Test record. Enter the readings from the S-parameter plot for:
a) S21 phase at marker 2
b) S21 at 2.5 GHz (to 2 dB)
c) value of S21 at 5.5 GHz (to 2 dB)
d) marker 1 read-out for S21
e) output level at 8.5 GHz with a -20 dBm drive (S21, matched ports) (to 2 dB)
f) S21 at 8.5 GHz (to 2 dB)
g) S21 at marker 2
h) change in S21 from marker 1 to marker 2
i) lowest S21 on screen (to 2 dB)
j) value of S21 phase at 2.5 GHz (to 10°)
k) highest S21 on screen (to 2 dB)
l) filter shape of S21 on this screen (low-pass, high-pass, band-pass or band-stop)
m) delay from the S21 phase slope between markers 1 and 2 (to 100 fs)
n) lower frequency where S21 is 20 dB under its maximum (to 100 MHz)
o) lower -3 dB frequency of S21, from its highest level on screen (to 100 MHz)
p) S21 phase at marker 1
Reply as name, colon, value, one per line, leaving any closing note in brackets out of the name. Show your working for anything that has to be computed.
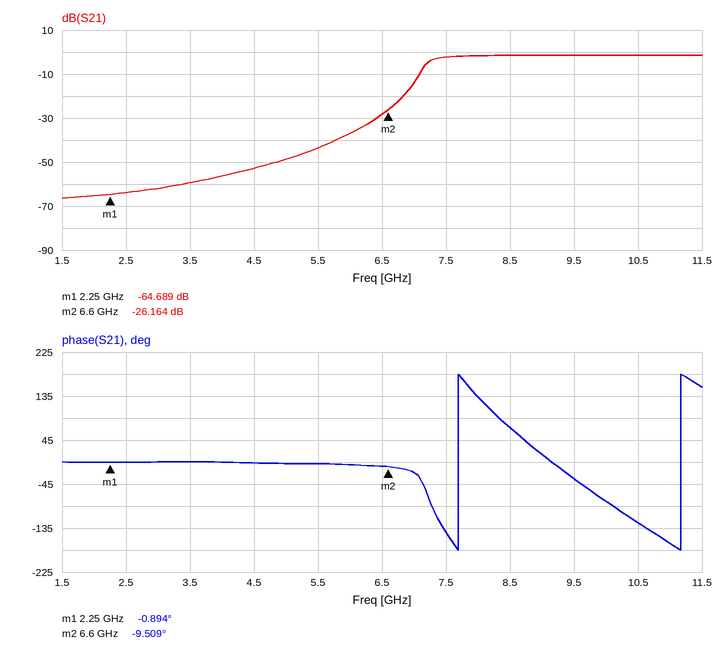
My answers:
S21 phase at marker 2: -9.509°
S21 at 2.5 GHz: -64 dB
value of S21 at 5.5 GHz: -44 dB
marker 1 read-out for S21: -64.689 dB
output level at 8.5 GHz with a -20 dBm drive (S21, matched ports): -20 dBm + (-2 dB) = -22 dBm
S21 at 8.5 GHz: -2 dB
S21 at marker 2: -26.164 dB
change in S21 from marker 1 to marker 2: -26.164 − (-64.689) = 38.525 dB
lowest S21 on screen: -66 dB
value of S21 phase at 2.5 GHz: 0°
highest S21 on screen: -2 dB
filter shape of S21 on this screen: high-pass
delay from the S21 phase slope between markers 1 and 2: −(-9.509° − (-0.894°))/(360° × 4.35 GHz) ≈ 5.5 ps
lower frequency where S21 is 20 dB under its maximum: 6.8 GHz
lower -3 dB frequency of S21, from its highest level on screen: 7.2 GHz
S21 phase at marker 1: -0.894°
